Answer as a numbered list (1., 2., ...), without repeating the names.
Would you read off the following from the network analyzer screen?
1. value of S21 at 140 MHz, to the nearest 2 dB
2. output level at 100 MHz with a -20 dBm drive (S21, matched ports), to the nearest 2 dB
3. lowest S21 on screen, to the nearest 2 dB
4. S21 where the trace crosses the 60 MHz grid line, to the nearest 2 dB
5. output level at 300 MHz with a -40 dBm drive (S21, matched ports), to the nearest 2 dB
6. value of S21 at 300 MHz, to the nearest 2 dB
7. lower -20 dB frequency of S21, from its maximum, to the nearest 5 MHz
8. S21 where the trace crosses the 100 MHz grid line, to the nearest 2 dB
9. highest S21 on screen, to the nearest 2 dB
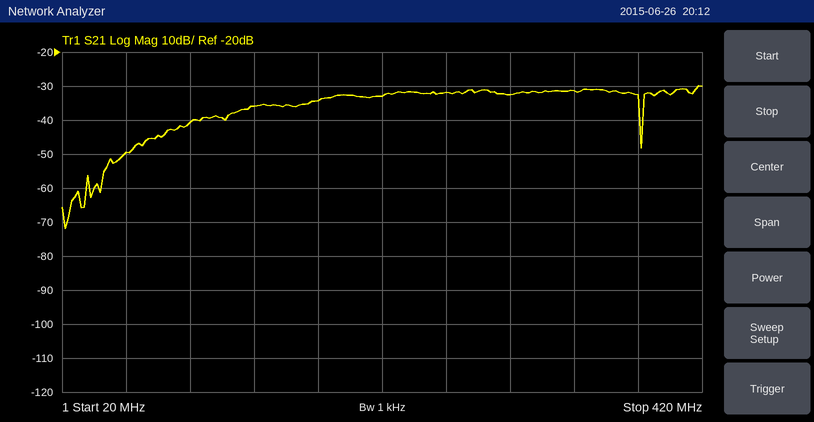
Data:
1. -36 dB
2. -60 dBm
3. -72 dB
4. -50 dB
5. -72 dBm
6. -32 dB
7. 60 MHz
8. -40 dB
9. -30 dB
